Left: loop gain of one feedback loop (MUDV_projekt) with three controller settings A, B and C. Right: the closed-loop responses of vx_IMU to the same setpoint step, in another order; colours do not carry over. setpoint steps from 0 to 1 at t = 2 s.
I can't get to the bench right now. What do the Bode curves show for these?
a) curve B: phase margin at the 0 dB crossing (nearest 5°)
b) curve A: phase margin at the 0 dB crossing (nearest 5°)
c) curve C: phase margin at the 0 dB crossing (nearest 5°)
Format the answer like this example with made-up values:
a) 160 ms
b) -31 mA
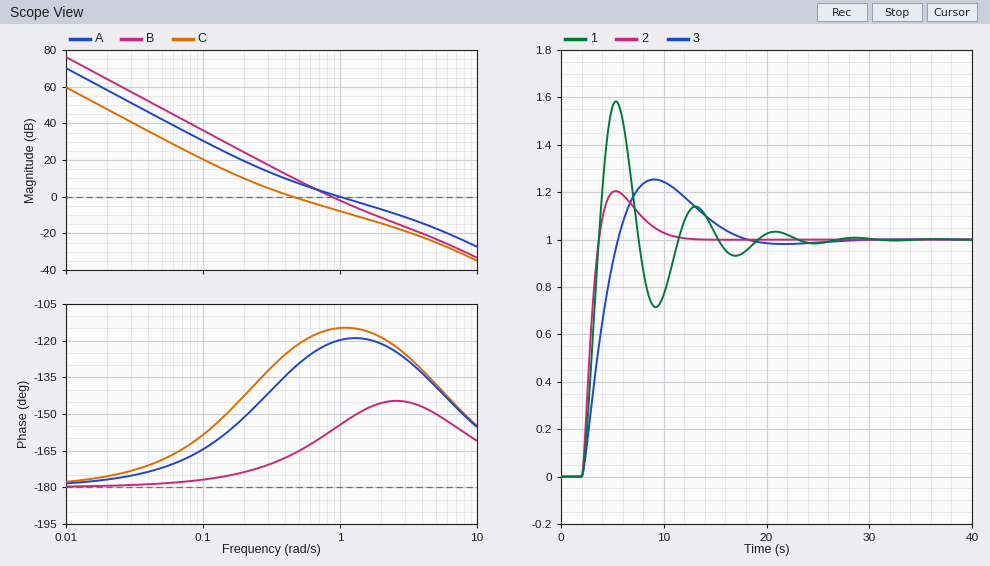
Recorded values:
a) 25°
b) 60°
c) 55°
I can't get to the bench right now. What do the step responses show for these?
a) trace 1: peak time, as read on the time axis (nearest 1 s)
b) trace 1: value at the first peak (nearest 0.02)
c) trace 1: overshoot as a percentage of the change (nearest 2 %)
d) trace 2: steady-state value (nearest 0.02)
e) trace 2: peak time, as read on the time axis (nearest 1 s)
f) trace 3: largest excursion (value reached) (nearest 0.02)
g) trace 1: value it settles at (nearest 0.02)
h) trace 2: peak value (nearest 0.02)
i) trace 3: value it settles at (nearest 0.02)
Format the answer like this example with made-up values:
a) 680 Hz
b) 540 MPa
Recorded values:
a) 5 s
b) 1.58
c) 58 %
d) 1.00
e) 5 s
f) 1.26
g) 1.00
h) 1.20
i) 1.00
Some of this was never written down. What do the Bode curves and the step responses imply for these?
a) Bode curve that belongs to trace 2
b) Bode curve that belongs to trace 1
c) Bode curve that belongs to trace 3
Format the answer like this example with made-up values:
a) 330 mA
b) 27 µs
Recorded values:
a) A
b) B
c) C
